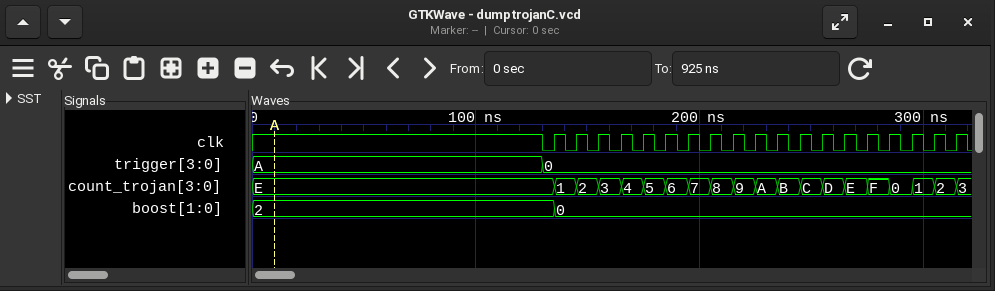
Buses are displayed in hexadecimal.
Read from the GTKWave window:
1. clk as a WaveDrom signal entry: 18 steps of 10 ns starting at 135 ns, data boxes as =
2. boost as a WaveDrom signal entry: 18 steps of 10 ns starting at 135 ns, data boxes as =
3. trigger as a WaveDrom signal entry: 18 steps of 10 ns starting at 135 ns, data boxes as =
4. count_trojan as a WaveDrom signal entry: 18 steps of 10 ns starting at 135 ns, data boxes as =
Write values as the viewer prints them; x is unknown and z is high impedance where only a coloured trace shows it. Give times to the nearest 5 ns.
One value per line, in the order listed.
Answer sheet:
{name: 'clk', wave: 'p.................'}
{name: 'boost', wave: '=.................', data: '0'}
{name: 'trigger', wave: '=.................', data: '0'}
{name: 'count_trojan', wave: '==================', data: '1 2 3 4 5 6 7 8 9 A B C D E F 0 1 2'}
